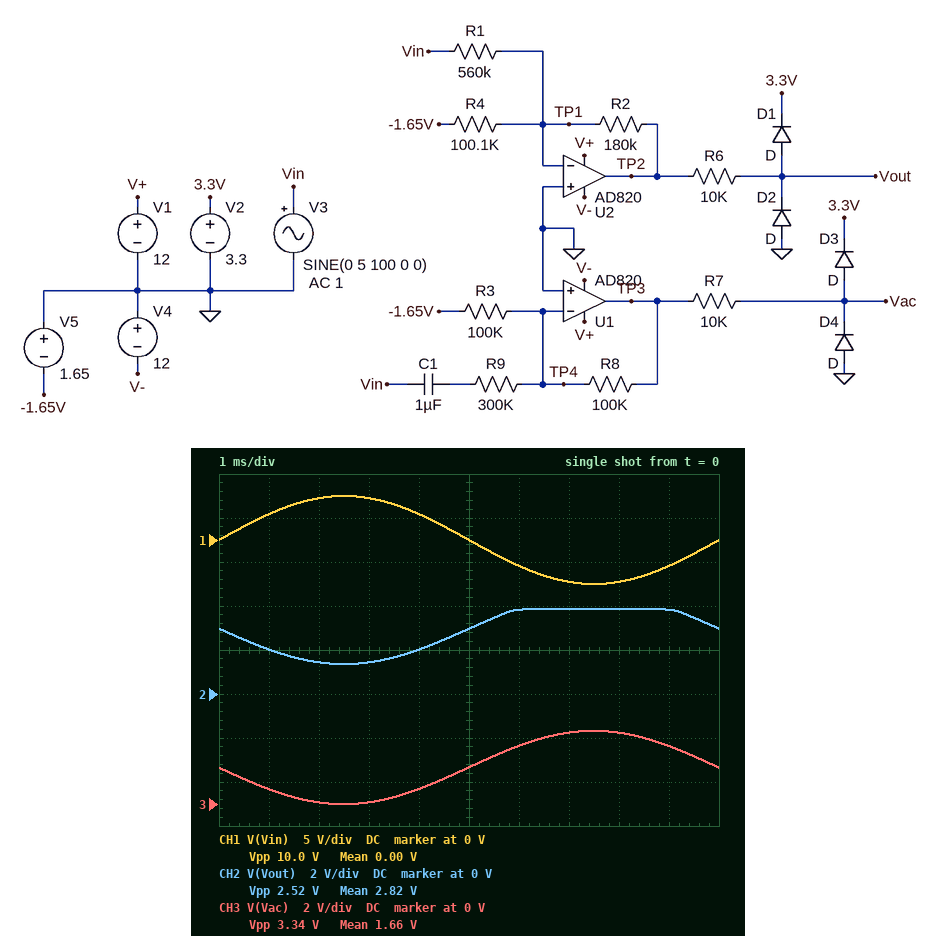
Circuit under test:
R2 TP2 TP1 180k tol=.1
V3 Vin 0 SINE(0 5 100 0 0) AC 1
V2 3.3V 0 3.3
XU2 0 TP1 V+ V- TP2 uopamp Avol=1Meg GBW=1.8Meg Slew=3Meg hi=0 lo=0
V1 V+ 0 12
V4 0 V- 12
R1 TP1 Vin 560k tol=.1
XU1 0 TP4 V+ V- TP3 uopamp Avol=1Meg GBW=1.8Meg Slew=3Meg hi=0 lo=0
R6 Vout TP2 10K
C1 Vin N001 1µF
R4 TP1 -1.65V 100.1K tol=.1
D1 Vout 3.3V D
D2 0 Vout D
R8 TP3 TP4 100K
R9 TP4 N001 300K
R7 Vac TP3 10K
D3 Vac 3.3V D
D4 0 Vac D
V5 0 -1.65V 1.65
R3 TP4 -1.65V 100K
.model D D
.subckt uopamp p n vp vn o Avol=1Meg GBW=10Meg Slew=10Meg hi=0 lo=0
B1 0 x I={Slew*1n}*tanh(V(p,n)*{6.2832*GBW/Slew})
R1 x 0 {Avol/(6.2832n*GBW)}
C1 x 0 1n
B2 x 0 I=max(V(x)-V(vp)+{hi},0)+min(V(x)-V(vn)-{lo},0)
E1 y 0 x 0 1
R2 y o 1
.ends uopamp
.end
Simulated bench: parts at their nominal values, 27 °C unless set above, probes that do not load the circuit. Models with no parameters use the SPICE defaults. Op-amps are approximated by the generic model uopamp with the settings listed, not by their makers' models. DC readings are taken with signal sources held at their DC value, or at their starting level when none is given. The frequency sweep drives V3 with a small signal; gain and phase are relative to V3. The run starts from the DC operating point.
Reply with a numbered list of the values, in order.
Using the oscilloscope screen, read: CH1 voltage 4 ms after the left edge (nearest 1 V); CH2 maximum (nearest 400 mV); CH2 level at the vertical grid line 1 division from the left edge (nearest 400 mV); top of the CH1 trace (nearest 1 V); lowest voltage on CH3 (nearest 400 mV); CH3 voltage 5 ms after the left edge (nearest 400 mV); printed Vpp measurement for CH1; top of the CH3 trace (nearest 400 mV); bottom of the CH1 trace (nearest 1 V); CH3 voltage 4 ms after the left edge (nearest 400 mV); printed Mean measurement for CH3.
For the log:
1. 3 V
2. 4.0 V
3. 2.0 V
4. 5 V
5. 0 V
6. 1.6 V
7. 10.0 V
8. 3.2 V
9. -5 V
10. 800 mV
11. 1.66 V
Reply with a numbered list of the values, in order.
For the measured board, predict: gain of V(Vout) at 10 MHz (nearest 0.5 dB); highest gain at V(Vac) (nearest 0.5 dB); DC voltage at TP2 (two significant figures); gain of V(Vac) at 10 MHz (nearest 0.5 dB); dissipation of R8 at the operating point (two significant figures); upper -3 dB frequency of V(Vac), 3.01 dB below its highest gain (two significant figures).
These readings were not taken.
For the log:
1. -34.5 dB
2. -9.5 dB
3. 3.0 V
4. -32.0 dB
5. 27 µW
6. 770 kHz
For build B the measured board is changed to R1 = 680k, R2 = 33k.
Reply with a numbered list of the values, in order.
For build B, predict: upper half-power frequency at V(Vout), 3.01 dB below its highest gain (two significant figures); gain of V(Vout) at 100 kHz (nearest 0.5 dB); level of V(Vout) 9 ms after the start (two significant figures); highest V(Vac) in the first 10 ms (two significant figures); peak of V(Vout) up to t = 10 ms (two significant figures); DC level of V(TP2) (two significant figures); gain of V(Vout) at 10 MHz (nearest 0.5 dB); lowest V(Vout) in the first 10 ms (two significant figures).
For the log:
1. 1.3 MHz
2. -26.5 dB
3. 690 mV
4. 3.3 V
5. 790 mV
6. 540 mV
7. -44.0 dB
8. 300 mV
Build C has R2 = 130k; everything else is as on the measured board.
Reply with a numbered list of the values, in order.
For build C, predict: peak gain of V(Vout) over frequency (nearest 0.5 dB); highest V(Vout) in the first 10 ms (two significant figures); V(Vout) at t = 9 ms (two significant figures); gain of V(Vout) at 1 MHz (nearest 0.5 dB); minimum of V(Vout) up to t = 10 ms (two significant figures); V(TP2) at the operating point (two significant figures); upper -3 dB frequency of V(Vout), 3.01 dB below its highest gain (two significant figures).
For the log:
1. -12.5 dB
2. 3.3 V
3. 2.8 V
4. -17.5 dB
5. 980 mV
6. 2.1 V
7. 710 kHz
